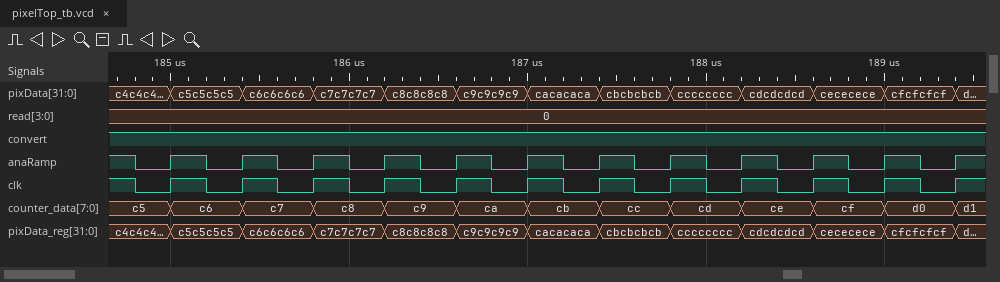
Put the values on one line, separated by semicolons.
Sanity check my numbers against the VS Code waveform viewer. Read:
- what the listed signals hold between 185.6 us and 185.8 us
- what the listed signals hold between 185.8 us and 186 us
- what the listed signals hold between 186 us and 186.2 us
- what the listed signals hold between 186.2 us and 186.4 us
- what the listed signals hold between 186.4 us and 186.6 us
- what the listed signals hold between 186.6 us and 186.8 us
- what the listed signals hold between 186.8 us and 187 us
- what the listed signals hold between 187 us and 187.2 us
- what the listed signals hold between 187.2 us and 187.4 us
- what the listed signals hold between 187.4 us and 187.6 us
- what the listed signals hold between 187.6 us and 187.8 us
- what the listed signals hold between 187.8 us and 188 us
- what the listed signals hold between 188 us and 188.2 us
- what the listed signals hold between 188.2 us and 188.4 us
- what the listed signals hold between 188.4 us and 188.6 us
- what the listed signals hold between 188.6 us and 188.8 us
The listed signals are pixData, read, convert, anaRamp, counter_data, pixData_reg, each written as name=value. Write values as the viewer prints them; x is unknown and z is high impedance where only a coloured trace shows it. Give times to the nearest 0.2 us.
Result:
pixData=c6c6c6c6, read=0, convert=1, anaRamp=0, counter_data=c7, pixData_reg=c6c6c6c6; pixData=c7c7c7c7, read=0, convert=1, anaRamp=1, counter_data=c8, pixData_reg=c7c7c7c7; pixData=c7c7c7c7, read=0, convert=1, anaRamp=0, counter_data=c8, pixData_reg=c7c7c7c7; pixData=c8c8c8c8, read=0, convert=1, anaRamp=1, counter_data=c9, pixData_reg=c8c8c8c8; pixData=c8c8c8c8, read=0, convert=1, anaRamp=0, counter_data=c9, pixData_reg=c8c8c8c8; pixData=c9c9c9c9, read=0, convert=1, anaRamp=1, counter_data=ca, pixData_reg=c9c9c9c9; pixData=c9c9c9c9, read=0, convert=1, anaRamp=0, counter_data=ca, pixData_reg=c9c9c9c9; pixData=cacacaca, read=0, convert=1, anaRamp=1, counter_data=cb, pixData_reg=cacacaca; pixData=cacacaca, read=0, convert=1, anaRamp=0, counter_data=cb, pixData_reg=cacacaca; pixData=cbcbcbcb, read=0, convert=1, anaRamp=1, counter_data=cc, pixData_reg=cbcbcbcb; pixData=cbcbcbcb, read=0, convert=1, anaRamp=0, counter_data=cc, pixData_reg=cbcbcbcb; pixData=cccccccc, read=0, convert=1, anaRamp=1, counter_data=cd, pixData_reg=cccccccc; pixData=cccccccc, read=0, convert=1, anaRamp=0, counter_data=cd, pixData_reg=cccccccc; pixData=cdcdcdcd, read=0, convert=1, anaRamp=1, counter_data=ce, pixData_reg=cdcdcdcd; pixData=cdcdcdcd, read=0, convert=1, anaRamp=0, counter_data=ce, pixData_reg=cdcdcdcd; pixData=cececece, read=0, convert=1, anaRamp=1, counter_data=cf, pixData_reg=cececece
